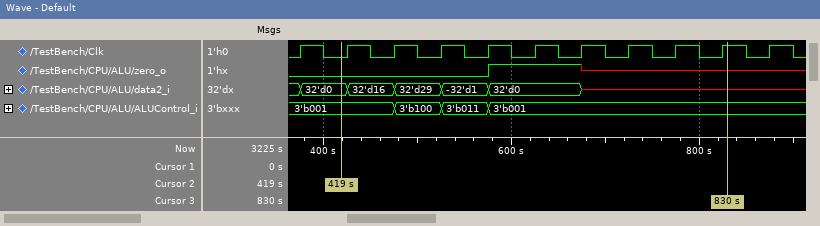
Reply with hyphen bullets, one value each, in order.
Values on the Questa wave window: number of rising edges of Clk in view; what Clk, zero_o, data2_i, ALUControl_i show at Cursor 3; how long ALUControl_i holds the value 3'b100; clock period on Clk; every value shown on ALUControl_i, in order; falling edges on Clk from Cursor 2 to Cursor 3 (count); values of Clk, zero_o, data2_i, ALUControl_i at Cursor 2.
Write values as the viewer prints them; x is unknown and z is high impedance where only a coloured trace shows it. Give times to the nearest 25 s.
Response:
- 11
- Clk=1, zero_o=x, data2_i=x, ALUControl_i=3'b001
- 50 s
- 50 s
- 3'b001, 3'b100, 3'b011, 3'b001
- 8
- Clk=0, zero_o=0, data2_i=32'd0, ALUControl_i=3'b001
